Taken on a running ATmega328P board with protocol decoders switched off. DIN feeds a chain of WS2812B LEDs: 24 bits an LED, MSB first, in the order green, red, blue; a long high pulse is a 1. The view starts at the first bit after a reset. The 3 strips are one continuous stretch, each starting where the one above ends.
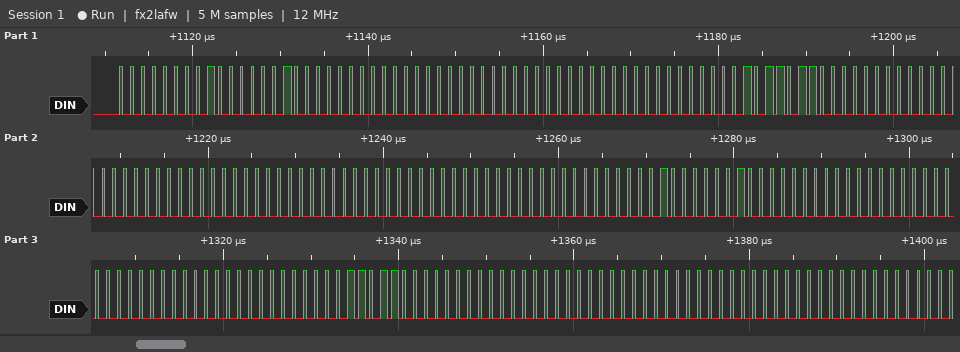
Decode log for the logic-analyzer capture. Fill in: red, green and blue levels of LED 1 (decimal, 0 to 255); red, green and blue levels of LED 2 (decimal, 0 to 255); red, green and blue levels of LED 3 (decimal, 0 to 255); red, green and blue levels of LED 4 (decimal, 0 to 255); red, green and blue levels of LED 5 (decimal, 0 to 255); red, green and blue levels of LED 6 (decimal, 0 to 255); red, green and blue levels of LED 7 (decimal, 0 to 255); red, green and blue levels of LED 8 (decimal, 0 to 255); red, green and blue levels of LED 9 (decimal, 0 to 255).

129, 0, 0
0, 0, 0
91, 0, 0
0, 0, 0
0, 0, 0
129, 0, 0
0, 0, 0
54, 0, 0
0, 0, 0
